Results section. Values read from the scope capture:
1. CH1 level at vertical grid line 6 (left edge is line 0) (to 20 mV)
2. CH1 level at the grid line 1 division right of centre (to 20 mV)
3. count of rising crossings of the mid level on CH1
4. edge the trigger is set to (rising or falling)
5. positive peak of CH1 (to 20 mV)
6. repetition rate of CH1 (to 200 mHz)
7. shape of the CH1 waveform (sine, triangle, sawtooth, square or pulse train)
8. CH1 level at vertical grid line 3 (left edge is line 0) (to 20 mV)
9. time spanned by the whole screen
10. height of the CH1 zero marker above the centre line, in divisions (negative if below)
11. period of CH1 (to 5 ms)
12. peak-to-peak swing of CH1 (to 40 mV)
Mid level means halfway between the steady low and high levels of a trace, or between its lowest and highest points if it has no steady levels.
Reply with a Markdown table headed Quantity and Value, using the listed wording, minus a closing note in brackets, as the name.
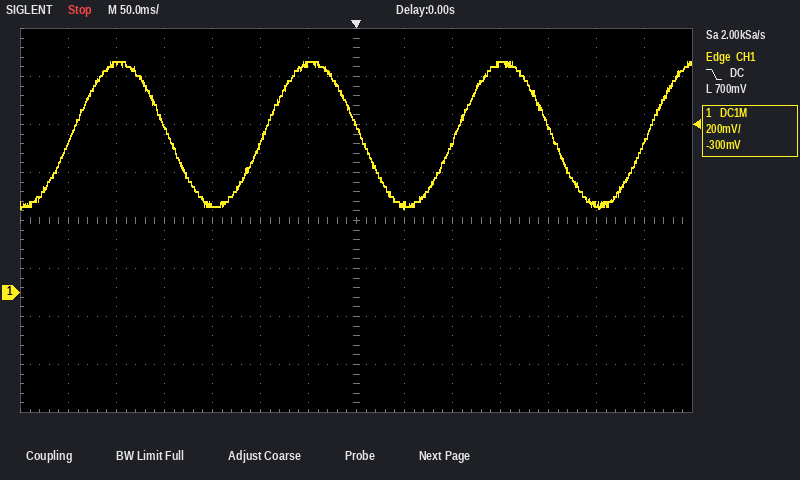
| Quantity | Value |
|---|---|
| CH1 level at vertical grid line 6 (left edge is line 0) | 960 mV |
| CH1 level at the grid line 1 division right of centre | 360 mV |
| count of rising crossings of the mid level on CH1 | 4 |
| edge the trigger is set to | falling |
| positive peak of CH1 | 960 mV |
| repetition rate of CH1 | 5.0 Hz |
| shape of the CH1 waveform | sine |
| CH1 level at vertical grid line 3 (left edge is line 0) | 700 mV |
| time spanned by the whole screen | 700 ms |
| height of the CH1 zero marker above the centre line, in divisions | -1.5 div |
| period of CH1 | 200 ms |
| peak-to-peak swing of CH1 | 600 mV |
